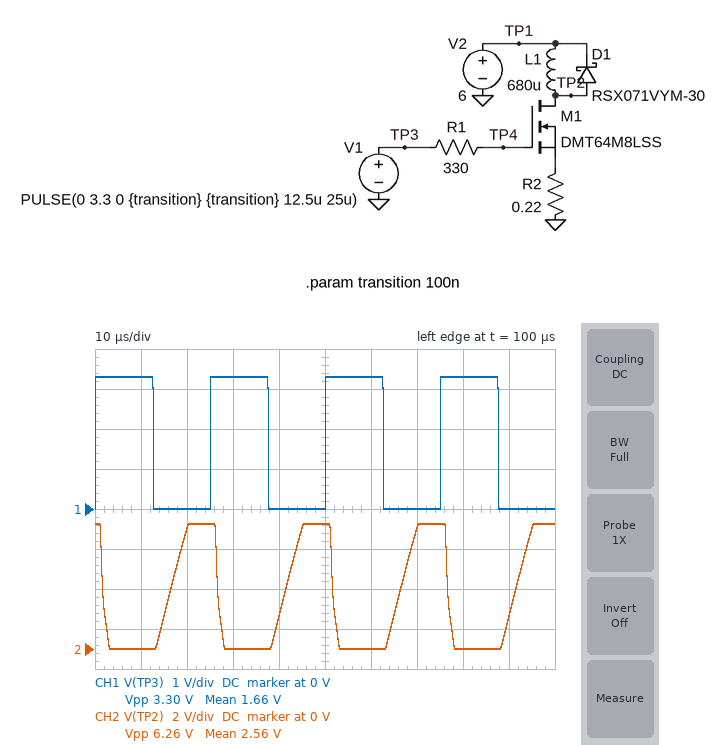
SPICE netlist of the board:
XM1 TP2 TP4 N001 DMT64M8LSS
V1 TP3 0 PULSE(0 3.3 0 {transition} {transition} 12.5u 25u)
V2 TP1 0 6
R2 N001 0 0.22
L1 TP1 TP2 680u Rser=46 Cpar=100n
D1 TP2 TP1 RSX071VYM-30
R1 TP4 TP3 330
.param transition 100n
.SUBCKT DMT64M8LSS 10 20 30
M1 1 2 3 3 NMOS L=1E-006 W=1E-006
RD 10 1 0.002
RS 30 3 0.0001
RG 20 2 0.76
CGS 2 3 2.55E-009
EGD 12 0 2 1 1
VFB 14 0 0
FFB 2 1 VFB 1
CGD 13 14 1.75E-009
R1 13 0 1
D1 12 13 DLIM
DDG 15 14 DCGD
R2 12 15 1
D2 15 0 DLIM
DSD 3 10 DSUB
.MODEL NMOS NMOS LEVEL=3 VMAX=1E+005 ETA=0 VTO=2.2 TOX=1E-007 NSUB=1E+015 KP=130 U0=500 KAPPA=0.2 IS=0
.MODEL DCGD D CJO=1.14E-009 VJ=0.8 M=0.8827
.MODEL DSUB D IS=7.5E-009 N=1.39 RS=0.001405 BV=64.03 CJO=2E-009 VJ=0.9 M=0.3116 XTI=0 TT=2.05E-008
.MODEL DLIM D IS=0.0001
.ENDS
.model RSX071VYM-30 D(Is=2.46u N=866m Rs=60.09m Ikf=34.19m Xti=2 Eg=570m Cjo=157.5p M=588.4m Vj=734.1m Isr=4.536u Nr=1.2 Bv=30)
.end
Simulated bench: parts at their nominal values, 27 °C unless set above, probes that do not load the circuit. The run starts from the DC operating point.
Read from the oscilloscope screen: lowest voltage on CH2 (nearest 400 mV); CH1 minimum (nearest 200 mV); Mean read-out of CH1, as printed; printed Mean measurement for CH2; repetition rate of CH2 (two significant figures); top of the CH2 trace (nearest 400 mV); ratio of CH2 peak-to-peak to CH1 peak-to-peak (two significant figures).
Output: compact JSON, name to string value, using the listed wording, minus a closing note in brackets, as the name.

{"lowest voltage on CH2": "0 V", "CH1 minimum": "0 V", "Mean read-out of CH1, as printed": "1.66 V", "printed Mean measurement for CH2": "2.56 V", "repetition rate of CH2": "40 kHz", "top of the CH2 trace": "6.4 V", "ratio of CH2 peak-to-peak to CH1 peak-to-peak": "1.9"}
